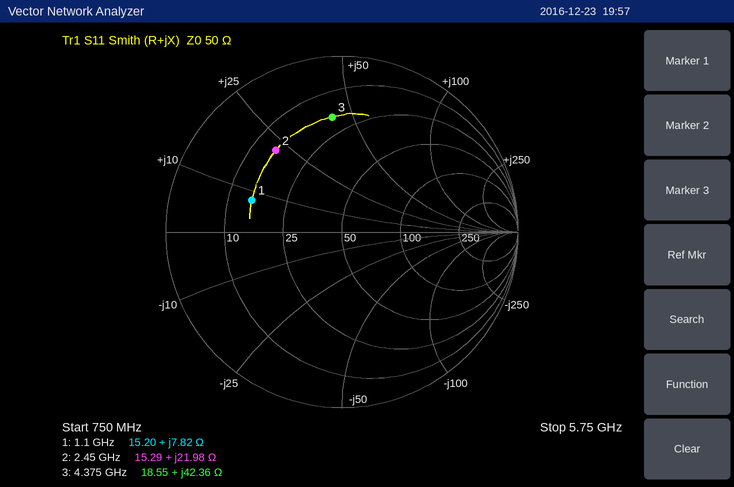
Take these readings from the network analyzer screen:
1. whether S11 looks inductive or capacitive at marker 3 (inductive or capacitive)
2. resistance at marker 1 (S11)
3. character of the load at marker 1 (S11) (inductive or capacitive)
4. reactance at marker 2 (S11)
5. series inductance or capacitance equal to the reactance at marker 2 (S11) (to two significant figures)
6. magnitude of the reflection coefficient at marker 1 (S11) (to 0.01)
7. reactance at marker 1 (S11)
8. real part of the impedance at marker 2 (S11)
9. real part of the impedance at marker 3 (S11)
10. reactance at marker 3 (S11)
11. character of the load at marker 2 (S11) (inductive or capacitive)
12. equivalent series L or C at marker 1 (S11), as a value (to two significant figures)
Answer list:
inductive
15.20 Ω
inductive
+21.98 Ω
1.4 nH
0.54
+7.82 Ω
15.29 Ω
18.55 Ω
+42.36 Ω
inductive
1.1 nH
